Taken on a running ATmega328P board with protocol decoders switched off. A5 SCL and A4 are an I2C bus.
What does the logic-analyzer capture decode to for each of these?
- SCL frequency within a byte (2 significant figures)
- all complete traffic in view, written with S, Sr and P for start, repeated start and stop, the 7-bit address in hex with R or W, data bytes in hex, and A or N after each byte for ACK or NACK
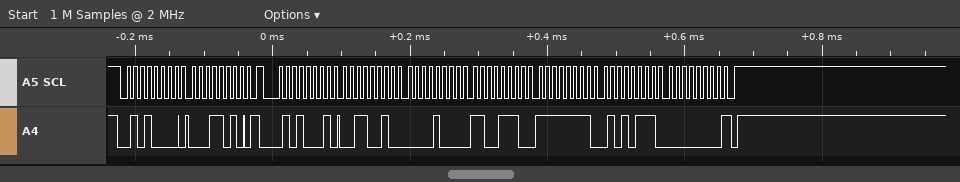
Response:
100 kHz
S 28W A 1A A Sr 28R A 32 A 08 A CE A FF A 57 A 00 N P
